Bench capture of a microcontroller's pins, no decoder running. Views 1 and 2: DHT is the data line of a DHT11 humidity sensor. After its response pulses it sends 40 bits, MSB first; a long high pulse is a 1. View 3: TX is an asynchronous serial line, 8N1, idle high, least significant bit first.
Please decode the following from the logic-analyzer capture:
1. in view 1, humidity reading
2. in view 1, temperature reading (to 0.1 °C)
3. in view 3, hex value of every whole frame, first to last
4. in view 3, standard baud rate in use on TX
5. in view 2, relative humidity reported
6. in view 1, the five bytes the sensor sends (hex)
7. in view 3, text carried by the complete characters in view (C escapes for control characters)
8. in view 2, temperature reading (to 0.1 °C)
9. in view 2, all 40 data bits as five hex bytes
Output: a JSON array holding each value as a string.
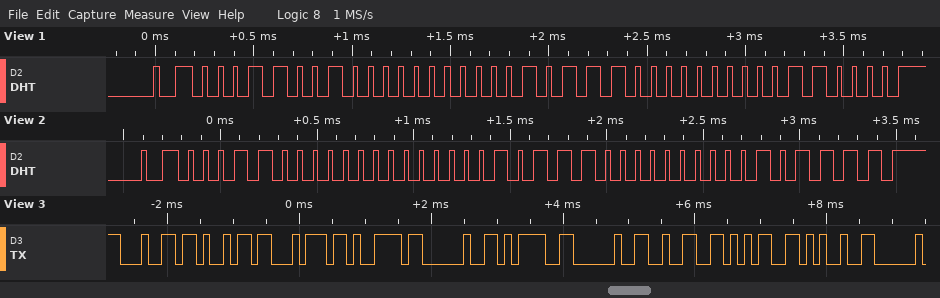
["25 %", "23.0 °C", "0x64 0x69 0x74 0x79 0x20 0x3D 0x20 0x32 0x35 0x25", "9600 baud", "24 %", "19 00 17 00 30", "\"dity = 25%\"", "23.0 °C", "18 00 17 00 2F"]
